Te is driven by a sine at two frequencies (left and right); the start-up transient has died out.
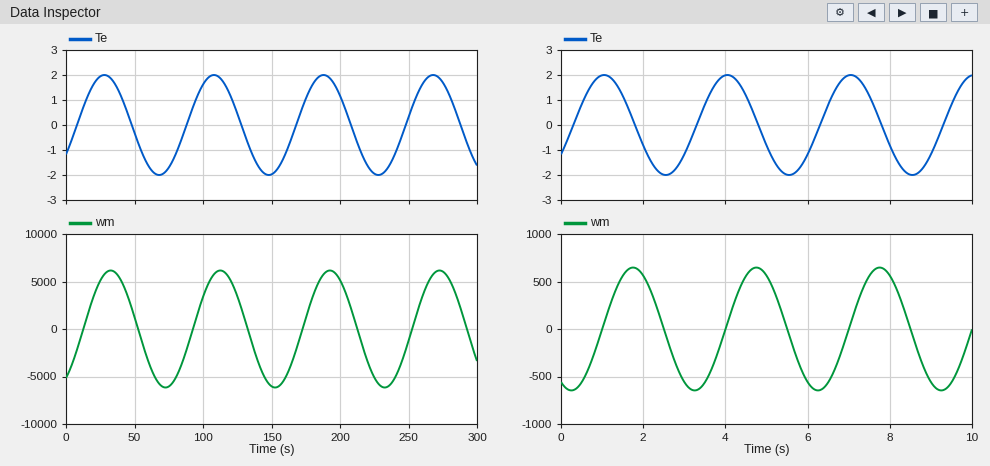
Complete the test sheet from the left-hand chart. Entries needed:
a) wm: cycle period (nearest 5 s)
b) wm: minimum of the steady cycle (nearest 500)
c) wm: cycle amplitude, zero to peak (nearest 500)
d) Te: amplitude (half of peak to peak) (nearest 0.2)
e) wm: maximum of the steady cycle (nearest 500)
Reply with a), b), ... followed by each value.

a) 80 s
b) -6000
c) 6000
d) 2.0
e) 6000
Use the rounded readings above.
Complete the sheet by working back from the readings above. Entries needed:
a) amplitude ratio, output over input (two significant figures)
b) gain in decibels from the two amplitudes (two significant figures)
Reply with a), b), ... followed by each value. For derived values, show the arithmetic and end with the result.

a) 6000 / 2 = 3000
b) 20 log10(6000 / 2) = 70 dB
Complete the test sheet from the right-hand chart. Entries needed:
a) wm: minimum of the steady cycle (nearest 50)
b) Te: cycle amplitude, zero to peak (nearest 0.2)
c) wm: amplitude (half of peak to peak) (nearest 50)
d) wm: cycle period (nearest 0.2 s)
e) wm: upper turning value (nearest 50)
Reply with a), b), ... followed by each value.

a) -650
b) 2.0
c) 650
d) 3.0 s
e) 650
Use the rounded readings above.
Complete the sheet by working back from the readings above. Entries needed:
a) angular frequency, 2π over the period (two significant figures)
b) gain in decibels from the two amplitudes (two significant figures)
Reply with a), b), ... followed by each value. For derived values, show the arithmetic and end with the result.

a) 2π / 3 = 2.1 rad/s
b) 20 log10(650 / 2) = 50 dB
